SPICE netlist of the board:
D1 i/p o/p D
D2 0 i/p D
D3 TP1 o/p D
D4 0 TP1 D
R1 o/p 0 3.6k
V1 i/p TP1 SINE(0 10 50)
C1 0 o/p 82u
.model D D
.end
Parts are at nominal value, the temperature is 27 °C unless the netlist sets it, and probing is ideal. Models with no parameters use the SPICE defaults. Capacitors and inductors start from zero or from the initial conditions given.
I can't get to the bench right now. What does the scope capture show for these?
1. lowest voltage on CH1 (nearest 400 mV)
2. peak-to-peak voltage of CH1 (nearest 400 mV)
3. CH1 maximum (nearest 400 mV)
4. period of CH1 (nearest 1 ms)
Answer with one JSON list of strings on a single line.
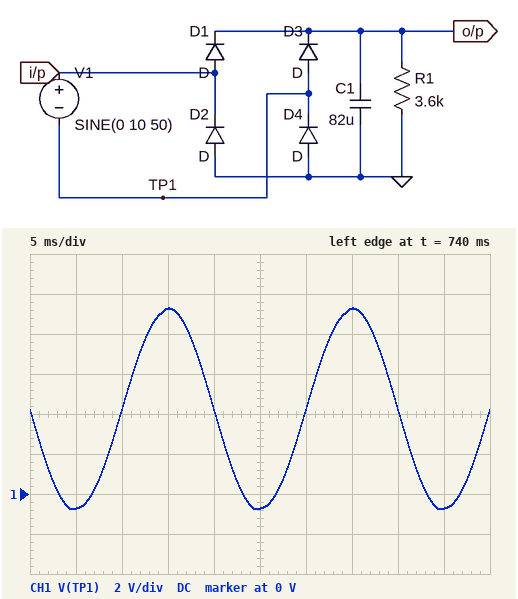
["-800 mV", "10.0 V", "9.2 V", "20 ms"]
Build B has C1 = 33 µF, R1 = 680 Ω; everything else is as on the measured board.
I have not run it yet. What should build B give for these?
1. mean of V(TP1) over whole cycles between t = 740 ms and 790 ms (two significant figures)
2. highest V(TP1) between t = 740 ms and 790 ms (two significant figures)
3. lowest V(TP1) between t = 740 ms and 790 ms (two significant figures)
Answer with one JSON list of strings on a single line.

["3.7 V", "9.3 V", "-770 mV"]
